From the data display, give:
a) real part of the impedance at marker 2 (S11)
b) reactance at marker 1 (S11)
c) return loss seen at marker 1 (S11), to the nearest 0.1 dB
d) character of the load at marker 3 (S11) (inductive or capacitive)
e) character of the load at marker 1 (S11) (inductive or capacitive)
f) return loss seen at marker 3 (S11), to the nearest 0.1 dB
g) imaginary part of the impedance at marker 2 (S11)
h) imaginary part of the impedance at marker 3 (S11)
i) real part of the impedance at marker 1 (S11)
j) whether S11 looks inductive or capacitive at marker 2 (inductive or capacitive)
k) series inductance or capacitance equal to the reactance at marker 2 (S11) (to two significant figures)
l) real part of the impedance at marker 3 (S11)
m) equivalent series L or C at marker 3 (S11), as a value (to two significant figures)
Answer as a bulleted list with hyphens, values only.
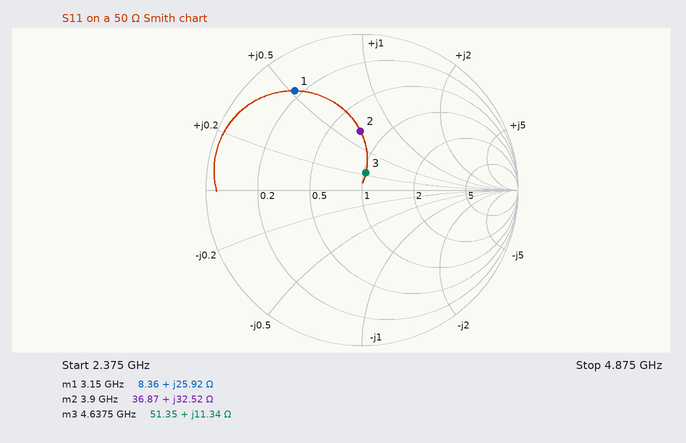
- 36.87 Ω
- +25.92 Ω
- 2.3 dB
- inductive
- inductive
- 19.0 dB
- +32.52 Ω
- +11.34 Ω
- 8.36 Ω
- inductive
- 1.3 nH
- 51.35 Ω
- 390 pH
